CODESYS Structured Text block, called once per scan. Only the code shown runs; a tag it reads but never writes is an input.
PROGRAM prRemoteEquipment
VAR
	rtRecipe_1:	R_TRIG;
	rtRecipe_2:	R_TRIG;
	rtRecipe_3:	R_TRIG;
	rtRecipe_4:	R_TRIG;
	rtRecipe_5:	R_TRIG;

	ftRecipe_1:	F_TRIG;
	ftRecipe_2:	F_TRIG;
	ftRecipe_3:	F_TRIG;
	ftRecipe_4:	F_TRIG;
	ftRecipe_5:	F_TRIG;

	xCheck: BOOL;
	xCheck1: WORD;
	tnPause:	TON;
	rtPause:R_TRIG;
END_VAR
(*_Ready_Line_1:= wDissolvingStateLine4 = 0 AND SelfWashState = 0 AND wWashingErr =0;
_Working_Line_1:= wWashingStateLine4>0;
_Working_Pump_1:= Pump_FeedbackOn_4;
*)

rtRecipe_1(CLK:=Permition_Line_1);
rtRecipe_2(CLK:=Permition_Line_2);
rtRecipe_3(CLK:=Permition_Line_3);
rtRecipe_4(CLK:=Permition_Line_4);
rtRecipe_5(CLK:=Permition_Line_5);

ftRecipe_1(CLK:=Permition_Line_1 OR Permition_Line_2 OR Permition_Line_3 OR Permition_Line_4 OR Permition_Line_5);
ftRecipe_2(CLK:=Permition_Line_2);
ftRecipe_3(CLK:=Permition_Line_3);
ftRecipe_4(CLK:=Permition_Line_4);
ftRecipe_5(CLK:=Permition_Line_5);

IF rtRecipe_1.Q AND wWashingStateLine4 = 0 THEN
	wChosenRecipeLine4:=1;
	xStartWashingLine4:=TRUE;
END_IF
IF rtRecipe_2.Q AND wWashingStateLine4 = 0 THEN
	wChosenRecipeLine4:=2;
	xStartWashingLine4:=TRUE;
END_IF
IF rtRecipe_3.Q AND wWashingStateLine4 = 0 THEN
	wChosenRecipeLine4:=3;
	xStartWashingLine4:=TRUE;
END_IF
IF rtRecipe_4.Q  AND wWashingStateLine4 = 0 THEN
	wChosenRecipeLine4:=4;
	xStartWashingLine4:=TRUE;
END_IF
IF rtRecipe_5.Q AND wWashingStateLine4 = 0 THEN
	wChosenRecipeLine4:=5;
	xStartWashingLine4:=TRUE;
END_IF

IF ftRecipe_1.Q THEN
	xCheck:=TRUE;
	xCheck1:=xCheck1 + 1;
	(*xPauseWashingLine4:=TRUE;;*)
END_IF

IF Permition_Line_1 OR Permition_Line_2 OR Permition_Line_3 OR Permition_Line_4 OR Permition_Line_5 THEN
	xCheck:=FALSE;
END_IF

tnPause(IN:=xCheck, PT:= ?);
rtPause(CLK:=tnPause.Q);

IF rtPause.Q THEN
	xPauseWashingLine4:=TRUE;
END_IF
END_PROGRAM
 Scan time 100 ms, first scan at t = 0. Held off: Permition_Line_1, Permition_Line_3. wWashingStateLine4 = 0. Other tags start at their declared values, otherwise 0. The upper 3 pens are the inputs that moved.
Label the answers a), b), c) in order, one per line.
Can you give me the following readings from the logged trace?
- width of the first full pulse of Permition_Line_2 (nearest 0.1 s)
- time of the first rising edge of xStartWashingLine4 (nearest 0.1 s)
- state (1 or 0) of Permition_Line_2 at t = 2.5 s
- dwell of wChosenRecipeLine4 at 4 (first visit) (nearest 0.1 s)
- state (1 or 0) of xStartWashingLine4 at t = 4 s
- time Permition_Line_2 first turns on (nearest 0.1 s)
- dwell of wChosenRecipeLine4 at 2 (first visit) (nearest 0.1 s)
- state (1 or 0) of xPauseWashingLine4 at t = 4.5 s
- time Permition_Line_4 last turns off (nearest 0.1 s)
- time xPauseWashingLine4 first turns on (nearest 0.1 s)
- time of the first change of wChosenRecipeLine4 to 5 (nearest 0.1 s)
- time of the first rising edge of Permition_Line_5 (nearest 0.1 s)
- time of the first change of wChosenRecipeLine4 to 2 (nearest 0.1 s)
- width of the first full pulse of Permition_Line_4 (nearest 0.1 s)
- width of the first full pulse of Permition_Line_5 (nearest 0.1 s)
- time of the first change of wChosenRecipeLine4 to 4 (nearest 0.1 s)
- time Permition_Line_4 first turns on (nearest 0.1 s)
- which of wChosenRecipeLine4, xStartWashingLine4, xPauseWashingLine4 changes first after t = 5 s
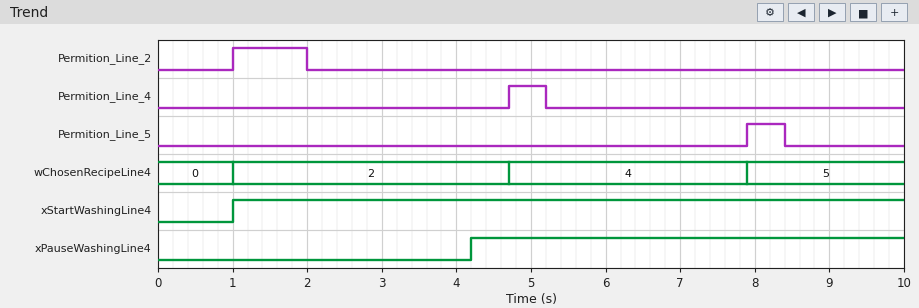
a) 1.0 s
b) 1.0 s
c) 0
d) 3.2 s
e) 1
f) 1.0 s
g) 3.7 s
h) 1
i) 5.2 s
j) 4.2 s
k) 7.9 s
l) 7.9 s
m) 1.0 s
n) 0.5 s
o) 0.5 s
p) 4.7 s
q) 4.7 s
r) wChosenRecipeLine4
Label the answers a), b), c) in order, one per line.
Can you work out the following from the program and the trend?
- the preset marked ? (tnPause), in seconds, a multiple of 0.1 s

a) 2.2 s
